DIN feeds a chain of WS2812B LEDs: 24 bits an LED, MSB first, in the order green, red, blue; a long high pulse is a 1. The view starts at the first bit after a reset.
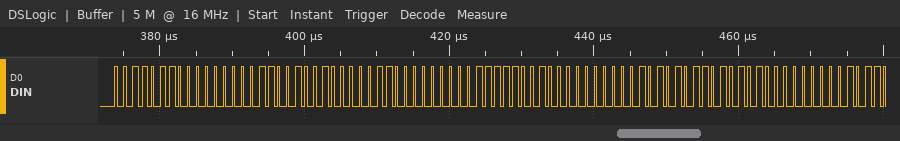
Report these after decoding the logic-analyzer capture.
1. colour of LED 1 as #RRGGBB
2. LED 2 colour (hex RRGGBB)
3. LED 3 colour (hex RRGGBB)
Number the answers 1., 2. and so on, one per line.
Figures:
1. #0036C9
2. #0006F9
3. #2A00D5
